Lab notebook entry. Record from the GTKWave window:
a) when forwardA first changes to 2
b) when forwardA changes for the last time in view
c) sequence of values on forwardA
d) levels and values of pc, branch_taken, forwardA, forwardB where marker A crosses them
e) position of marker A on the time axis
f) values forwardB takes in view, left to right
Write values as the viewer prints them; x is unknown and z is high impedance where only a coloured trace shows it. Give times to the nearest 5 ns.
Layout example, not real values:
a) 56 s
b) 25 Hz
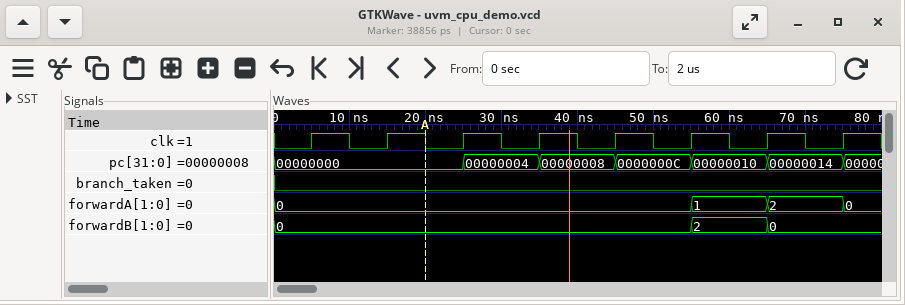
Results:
a) 65 ns
b) 75 ns
c) 0, 1, 2, 0
d) pc=00000000, branch_taken=0, forwardA=0, forwardB=0
e) 20 ns
f) 0, 2, 0
